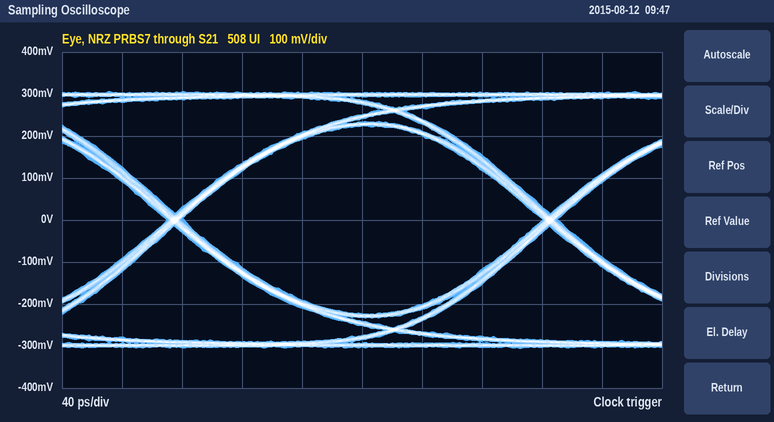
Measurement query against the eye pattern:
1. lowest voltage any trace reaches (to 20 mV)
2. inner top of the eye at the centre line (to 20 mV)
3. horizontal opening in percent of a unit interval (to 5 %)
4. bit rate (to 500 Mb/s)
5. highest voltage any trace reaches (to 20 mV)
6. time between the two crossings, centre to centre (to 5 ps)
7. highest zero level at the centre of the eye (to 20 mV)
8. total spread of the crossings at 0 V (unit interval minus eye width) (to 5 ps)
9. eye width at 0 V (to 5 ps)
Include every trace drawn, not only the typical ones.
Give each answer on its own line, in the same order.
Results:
-300 mV
220 mV
95 %
4.0 Gb/s
300 mV
250 ps
-220 mV
10 ps
240 ps
